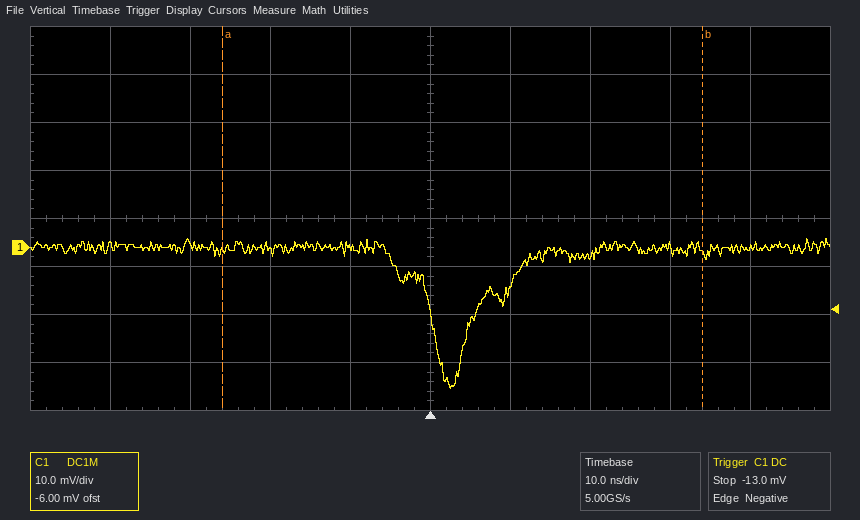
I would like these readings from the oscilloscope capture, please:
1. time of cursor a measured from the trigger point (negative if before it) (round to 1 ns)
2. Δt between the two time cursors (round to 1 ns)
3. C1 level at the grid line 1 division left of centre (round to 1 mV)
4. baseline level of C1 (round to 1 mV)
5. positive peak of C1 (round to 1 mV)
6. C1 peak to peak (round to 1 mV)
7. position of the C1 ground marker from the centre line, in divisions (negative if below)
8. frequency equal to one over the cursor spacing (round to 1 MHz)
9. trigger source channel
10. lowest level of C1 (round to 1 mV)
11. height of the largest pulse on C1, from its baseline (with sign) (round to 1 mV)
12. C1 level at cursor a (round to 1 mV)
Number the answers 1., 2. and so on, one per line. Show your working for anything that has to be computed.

1. -26 ns
2. 60 ns
3. 0 mV
4. 0 mV
5. 2 mV
6. 2 mV − (-29 mV) = 31 mV
7. -0.6 div
8. 1 / 60 ns ≈ 17 MHz
9. C1
10. -29 mV
11. -29 mV − (0 mV) = -29 mV
12. -1 mV
